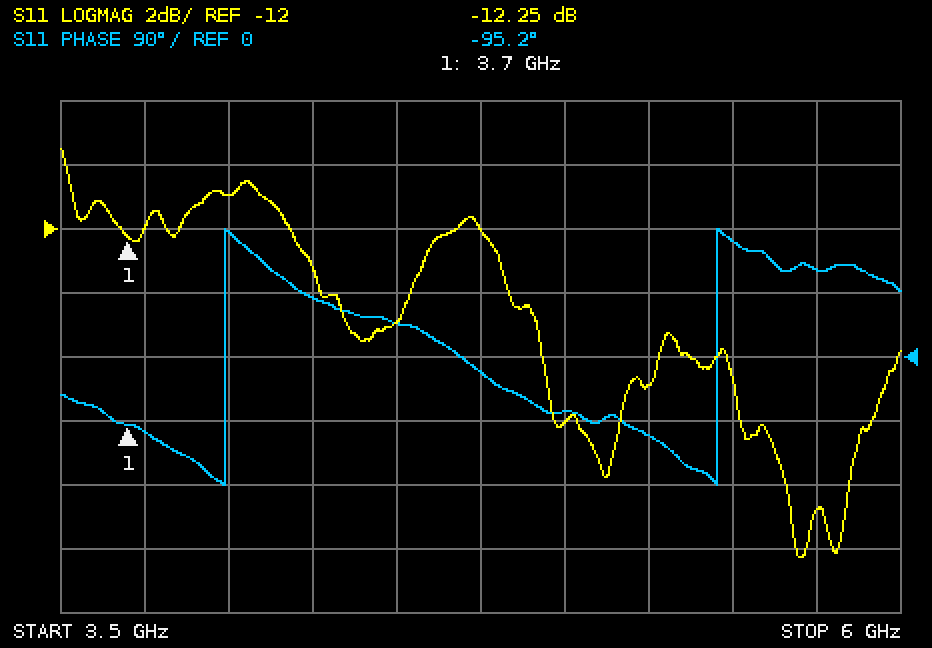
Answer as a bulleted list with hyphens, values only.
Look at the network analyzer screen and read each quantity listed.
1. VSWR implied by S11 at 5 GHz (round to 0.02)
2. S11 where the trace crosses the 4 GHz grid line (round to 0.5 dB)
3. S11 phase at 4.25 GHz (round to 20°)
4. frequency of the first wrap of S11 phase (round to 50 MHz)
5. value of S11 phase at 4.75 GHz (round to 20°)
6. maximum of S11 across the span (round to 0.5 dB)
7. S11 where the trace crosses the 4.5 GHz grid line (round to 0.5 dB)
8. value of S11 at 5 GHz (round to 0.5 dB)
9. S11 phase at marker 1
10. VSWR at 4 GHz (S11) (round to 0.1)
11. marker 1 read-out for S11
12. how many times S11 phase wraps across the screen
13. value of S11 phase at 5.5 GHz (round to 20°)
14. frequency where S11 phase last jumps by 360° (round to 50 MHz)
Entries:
- 1.28
- -11.0 dB
- 80°
- 4.00 GHz
- -20°
- -9.5 dB
- -15.0 dB
- -18.0 dB
- -95.2°
- 1.8
- -12.25 dB
- 2
- 160°
- 5.45 GHz
